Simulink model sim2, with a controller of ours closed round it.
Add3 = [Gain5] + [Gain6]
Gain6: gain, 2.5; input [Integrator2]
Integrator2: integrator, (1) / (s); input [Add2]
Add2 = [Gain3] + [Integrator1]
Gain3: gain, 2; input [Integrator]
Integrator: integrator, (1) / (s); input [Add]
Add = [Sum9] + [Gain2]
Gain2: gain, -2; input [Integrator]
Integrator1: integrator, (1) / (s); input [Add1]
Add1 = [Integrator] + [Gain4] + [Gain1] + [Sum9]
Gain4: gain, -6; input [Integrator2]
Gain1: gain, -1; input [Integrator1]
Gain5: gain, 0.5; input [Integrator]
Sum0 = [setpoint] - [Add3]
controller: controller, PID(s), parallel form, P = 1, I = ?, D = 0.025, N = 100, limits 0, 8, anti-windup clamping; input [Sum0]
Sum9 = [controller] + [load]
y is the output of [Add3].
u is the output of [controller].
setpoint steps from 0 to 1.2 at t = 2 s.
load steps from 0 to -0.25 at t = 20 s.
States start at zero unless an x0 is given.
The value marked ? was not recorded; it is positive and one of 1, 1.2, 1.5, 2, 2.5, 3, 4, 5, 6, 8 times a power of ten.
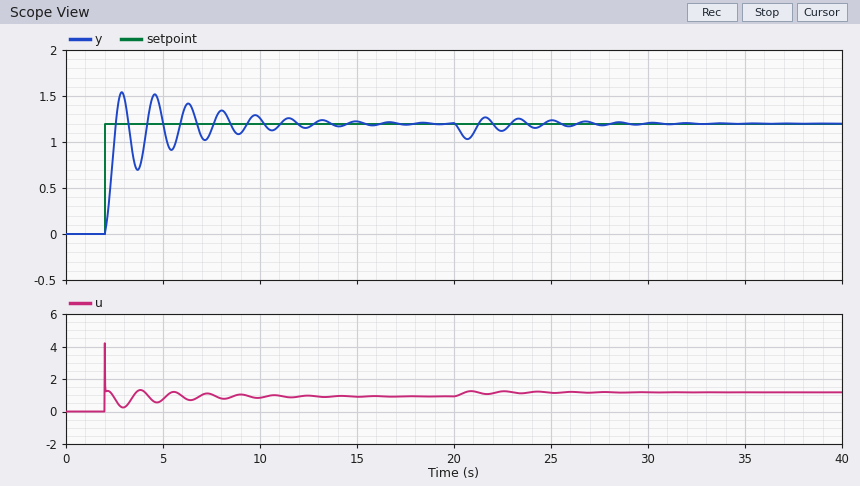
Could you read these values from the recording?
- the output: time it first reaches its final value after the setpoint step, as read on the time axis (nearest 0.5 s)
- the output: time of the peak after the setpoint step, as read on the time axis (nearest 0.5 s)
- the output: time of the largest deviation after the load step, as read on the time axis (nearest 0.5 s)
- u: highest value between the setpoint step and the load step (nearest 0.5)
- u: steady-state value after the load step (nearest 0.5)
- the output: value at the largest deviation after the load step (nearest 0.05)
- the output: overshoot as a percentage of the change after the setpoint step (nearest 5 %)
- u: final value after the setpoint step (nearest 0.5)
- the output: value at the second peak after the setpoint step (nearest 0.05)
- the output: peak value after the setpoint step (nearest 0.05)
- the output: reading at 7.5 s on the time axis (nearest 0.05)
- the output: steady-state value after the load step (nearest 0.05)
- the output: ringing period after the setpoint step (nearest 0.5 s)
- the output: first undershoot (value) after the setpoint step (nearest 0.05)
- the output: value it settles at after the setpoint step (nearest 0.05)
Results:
2.5 s
3.0 s
20.5 s
4.0
1.0
1.05
30 %
1.0
1.50
1.55
1.15
1.20
1.5 s
0.70
1.20
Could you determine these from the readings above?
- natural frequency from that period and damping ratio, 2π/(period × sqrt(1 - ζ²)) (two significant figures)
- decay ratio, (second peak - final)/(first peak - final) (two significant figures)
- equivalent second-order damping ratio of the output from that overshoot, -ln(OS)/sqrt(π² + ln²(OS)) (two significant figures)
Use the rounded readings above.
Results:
4.5 rad/s
0.86
0.36
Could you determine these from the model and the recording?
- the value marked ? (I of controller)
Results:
2
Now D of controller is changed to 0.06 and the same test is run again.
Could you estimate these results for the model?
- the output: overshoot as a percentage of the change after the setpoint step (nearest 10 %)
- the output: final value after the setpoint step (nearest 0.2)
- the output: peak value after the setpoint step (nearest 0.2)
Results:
20 %
1.2
1.4
